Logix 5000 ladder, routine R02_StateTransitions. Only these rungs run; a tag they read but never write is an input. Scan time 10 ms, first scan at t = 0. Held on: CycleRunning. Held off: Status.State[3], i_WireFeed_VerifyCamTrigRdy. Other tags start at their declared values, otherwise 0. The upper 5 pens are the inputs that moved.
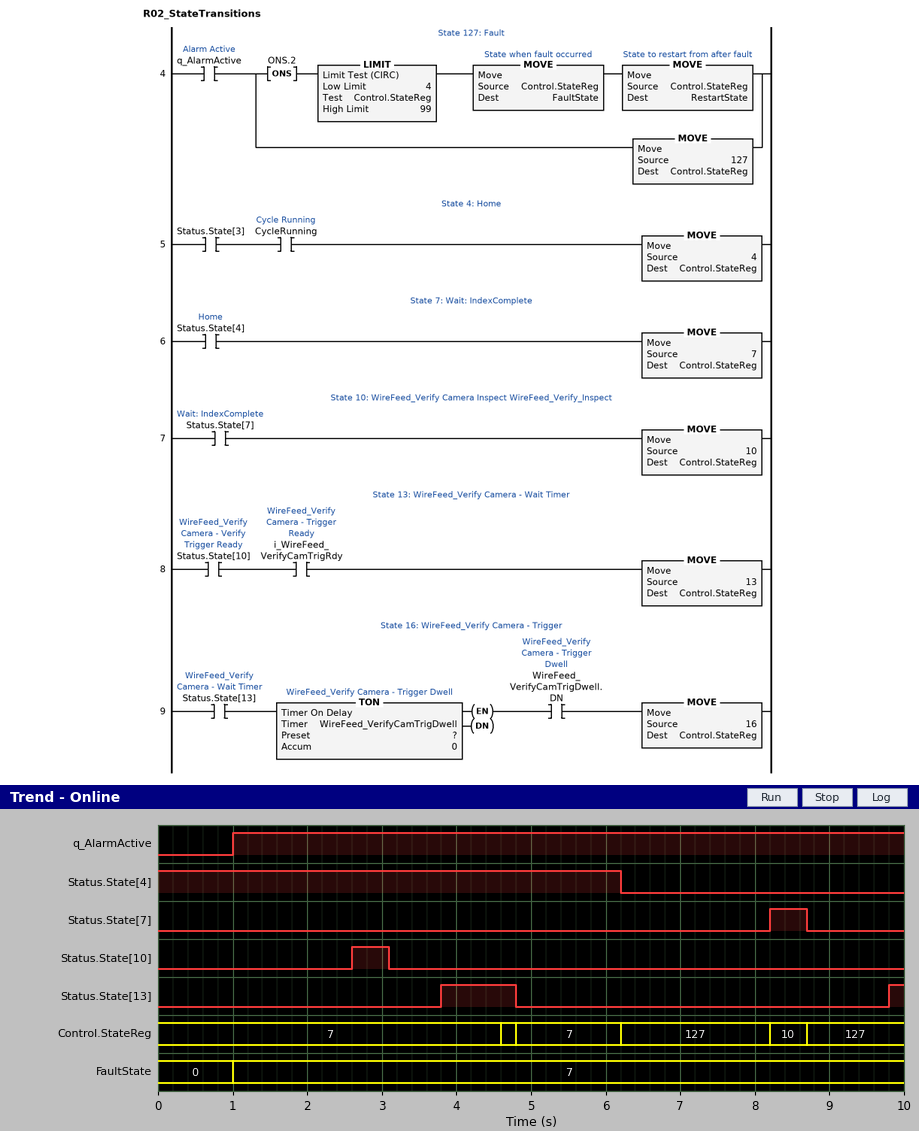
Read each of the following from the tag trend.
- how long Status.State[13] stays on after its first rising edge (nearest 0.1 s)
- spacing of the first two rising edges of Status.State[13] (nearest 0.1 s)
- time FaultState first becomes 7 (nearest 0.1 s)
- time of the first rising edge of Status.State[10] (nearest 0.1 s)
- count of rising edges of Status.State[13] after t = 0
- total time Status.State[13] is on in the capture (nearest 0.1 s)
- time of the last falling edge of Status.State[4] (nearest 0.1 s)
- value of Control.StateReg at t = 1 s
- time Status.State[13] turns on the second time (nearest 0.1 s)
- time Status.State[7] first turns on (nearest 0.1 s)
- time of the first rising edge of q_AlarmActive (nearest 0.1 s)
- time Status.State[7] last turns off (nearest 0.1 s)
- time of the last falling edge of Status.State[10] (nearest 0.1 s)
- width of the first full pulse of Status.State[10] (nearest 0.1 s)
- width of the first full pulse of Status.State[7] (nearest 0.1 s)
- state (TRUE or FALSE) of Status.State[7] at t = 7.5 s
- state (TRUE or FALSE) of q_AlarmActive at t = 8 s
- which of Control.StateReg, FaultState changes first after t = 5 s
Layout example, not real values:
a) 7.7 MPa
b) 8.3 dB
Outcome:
a) 1.0 s
b) 6.0 s
c) 1.0 s
d) 2.6 s
e) 2
f) 1.2 s
g) 6.2 s
h) 7
i) 9.8 s
j) 8.2 s
k) 1.0 s
l) 8.7 s
m) 3.1 s
n) 0.5 s
o) 0.5 s
p) FALSE
q) TRUE
r) Control.StateReg
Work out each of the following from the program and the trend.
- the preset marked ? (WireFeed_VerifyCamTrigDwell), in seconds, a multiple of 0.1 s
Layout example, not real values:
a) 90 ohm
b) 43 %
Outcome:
a) 0.8 s
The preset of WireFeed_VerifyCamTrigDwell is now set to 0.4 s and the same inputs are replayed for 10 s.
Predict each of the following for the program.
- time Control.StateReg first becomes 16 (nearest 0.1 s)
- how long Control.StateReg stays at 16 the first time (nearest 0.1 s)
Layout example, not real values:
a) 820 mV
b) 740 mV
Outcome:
a) 4.2 s
b) 0.6 s
